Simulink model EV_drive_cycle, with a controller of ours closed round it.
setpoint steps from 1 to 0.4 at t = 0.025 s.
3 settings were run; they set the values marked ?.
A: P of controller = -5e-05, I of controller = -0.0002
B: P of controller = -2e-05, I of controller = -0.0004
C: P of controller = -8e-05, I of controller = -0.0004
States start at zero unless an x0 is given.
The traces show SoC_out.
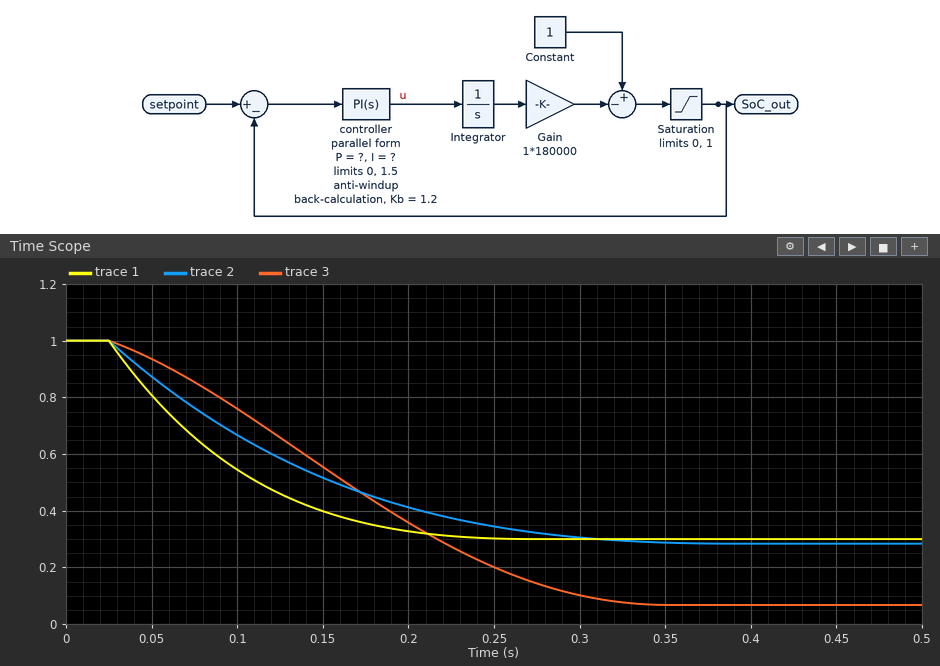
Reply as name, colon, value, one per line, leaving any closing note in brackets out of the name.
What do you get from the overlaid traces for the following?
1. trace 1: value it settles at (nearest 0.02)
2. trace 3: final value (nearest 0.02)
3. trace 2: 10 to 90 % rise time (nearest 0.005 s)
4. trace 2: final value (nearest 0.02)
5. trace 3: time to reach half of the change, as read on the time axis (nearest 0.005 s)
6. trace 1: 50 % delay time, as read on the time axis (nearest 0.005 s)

trace 1: value it settles at: 0.30
trace 3: final value: 0.06
trace 2: 10 to 90 % rise time: 0.200 s
trace 2: final value: 0.28
trace 3: time to reach half of the change, as read on the time axis: 0.155 s
trace 1: 50 % delay time, as read on the time axis: 0.075 s
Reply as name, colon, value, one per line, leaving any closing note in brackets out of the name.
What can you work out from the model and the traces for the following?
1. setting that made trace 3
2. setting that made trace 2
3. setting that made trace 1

setting that made trace 3: B
setting that made trace 2: A
setting that made trace 1: C
